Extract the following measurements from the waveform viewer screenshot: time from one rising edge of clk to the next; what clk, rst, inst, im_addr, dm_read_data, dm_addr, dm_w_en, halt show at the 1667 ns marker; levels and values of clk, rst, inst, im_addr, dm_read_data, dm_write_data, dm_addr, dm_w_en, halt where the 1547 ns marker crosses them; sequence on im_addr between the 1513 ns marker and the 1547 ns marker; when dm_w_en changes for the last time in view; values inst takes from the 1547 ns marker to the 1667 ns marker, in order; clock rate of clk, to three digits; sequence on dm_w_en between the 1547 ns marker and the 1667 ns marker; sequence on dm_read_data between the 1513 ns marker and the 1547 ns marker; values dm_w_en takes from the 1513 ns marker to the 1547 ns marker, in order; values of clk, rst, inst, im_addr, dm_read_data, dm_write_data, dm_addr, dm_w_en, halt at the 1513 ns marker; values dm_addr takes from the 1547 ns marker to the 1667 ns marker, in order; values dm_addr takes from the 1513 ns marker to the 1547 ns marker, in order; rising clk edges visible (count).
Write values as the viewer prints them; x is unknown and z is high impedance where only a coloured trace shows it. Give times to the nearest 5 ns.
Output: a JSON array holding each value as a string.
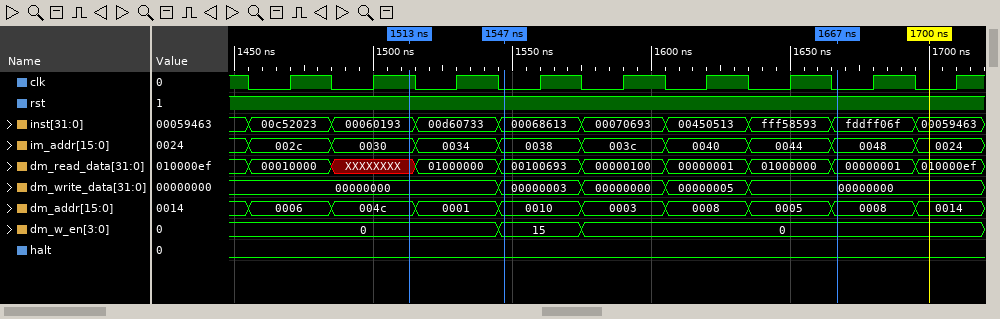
["30 ns", "clk=0, rst=1, inst=fddff06f, im_addr=0048, dm_read_data=00000001, dm_addr=0008, dm_w_en=0, halt=0", "clk=0, rst=1, inst=00068613, im_addr=0038, dm_read_data=00100693, dm_write_data=00000003, dm_addr=0010, dm_w_en=15, halt=0", "0030, 0034, 0038", "1575 ns", "00068613, 00070693, 00450513, fff58593, fddff06f", "33.3 MHz", "15, 0", "XXXXXXXX, 01000000, 00100693", "0, 15", "clk=1, rst=1, inst=00060193, im_addr=0030, dm_read_data=XXXXXXXX, dm_write_data=00000000, dm_addr=004c, dm_w_en=0, halt=0", "0010, 0003, 0008, 0005, 0008", "004c, 0001, 0010", "9"]
